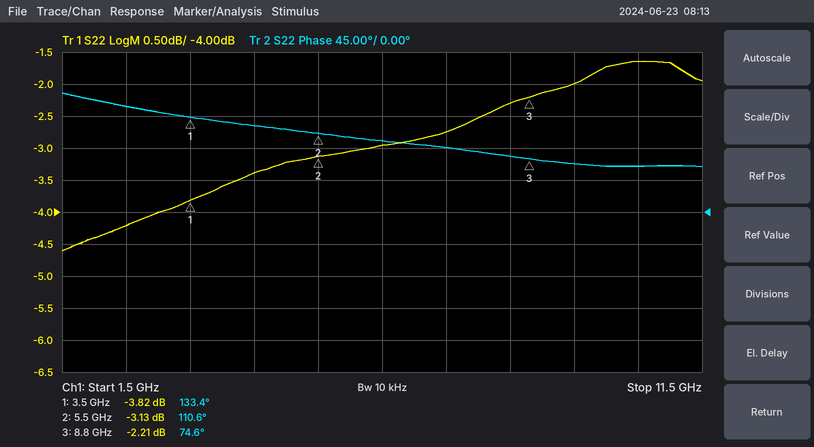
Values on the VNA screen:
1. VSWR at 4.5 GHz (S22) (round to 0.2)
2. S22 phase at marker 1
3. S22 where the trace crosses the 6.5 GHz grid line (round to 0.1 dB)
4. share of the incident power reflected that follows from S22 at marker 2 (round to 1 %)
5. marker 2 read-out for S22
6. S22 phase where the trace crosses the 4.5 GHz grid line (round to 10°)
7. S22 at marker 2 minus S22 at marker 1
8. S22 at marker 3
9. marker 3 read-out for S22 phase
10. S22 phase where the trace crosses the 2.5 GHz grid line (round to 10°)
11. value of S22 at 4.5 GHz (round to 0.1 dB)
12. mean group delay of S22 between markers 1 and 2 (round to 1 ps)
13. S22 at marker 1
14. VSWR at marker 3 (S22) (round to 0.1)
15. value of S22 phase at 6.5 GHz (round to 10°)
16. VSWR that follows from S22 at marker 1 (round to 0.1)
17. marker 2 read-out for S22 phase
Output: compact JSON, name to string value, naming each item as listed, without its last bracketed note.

{"VSWR at 4.5 GHz (S22)": "5.2", "S22 phase at marker 1": "133.4°", "S22 where the trace crosses the 6.5 GHz grid line": "-3.0 dB", "share of the incident power reflected that follows from S22 at marker 2": "49 %", "marker 2 read-out for S22": "-3.13 dB", "S22 phase where the trace crosses the 4.5 GHz grid line": "120°", "S22 at marker 2 minus S22 at marker 1": "0.69 dB", "S22 at marker 3": "-2.21 dB", "marker 3 read-out for S22 phase": "74.6°", "S22 phase where the trace crosses the 2.5 GHz grid line": "150°", "value of S22 at 4.5 GHz": "-3.4 dB", "mean group delay of S22 between markers 1 and 2": "32 ps", "S22 at marker 1": "-3.82 dB", "VSWR at marker 3 (S22)": "7.9", "value of S22 phase at 6.5 GHz": "100°", "VSWR that follows from S22 at marker 1": "4.6", "marker 2 read-out for S22 phase": "110.6°"}
